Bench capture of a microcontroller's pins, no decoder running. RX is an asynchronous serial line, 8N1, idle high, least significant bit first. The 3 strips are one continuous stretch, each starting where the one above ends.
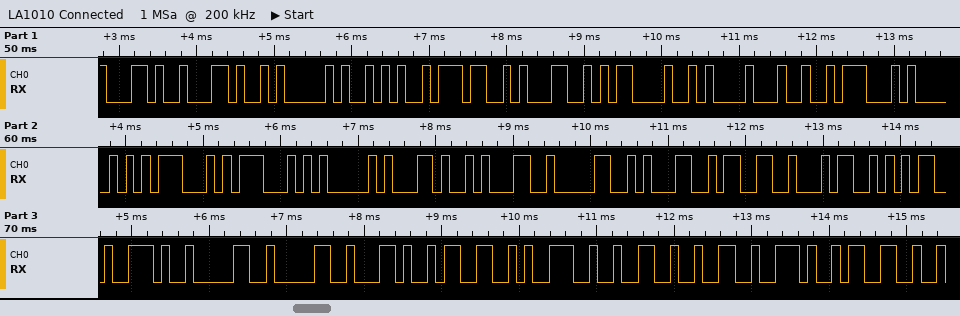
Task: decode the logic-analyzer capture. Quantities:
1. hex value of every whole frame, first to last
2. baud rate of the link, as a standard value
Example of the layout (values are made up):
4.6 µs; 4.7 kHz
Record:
2C 2C 41 2A 37 31 0D 0A 24 47 50 47 47 41 2C 31 30 31 33 34 35 2E 30 30 2C 33 39 32 32 2E 33; 9600 baud
